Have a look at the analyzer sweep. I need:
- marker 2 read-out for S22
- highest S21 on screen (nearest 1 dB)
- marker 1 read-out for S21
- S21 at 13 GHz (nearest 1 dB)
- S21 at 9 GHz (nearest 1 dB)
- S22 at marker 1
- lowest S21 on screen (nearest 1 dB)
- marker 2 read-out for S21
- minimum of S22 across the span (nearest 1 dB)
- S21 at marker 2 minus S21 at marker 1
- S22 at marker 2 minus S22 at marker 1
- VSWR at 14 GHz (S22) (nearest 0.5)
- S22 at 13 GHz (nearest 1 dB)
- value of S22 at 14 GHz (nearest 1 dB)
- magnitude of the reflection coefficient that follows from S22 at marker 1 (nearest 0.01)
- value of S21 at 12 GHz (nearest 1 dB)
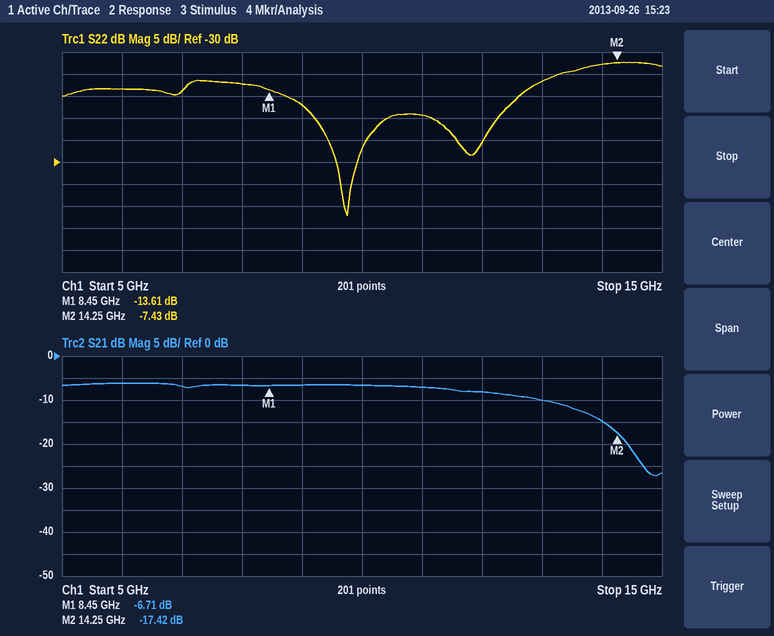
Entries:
-7.43 dB
-6 dB
-6.71 dB
-10 dB
-7 dB
-13.61 dB
-27 dB
-17.42 dB
-42 dB
-10.71 dB
6.18 dB
2.5
-12 dB
-8 dB
0.21
-8 dB
